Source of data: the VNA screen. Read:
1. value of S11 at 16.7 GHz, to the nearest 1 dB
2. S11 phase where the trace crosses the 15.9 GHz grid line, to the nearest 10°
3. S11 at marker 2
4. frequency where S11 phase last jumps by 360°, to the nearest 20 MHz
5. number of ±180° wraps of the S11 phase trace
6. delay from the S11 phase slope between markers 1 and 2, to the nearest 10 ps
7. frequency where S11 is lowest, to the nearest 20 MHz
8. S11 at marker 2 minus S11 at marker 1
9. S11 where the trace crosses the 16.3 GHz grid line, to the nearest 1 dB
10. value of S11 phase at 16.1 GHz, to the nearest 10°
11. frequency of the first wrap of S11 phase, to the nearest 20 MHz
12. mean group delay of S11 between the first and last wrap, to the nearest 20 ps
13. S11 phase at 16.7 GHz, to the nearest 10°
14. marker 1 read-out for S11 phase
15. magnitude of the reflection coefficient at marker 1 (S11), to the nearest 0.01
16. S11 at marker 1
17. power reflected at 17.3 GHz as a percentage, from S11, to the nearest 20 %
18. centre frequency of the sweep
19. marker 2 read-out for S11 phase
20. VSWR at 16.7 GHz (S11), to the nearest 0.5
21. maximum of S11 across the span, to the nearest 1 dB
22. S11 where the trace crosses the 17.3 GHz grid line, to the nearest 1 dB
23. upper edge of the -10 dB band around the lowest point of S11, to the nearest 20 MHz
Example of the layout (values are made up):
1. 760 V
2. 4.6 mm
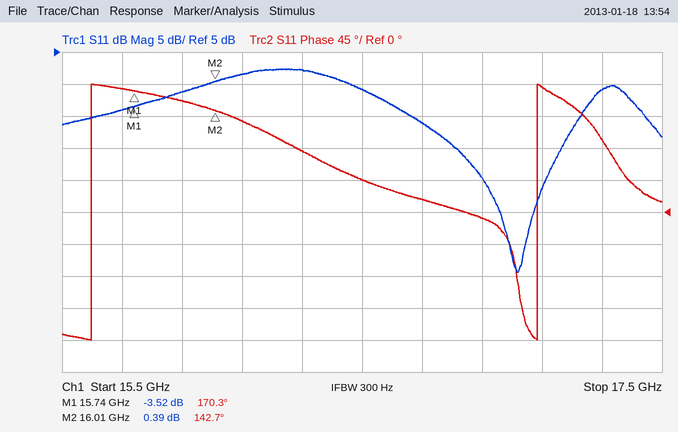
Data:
1. -6 dB
2. 160°
3. 0.39 dB
4. 17.08 GHz
5. 2
6. 280 ps
7. 17.02 GHz
8. 3.91 dB
9. 2 dB
10. 130°
11. 15.60 GHz
12. 680 ps
13. 20°
14. 170.3°
15. 0.67
16. -3.52 dB
17. 80 %
18. 16.5 GHz
19. 142.7°
20. 3.0
21. 2 dB
22. -1 dB
23. 17.16 GHz
